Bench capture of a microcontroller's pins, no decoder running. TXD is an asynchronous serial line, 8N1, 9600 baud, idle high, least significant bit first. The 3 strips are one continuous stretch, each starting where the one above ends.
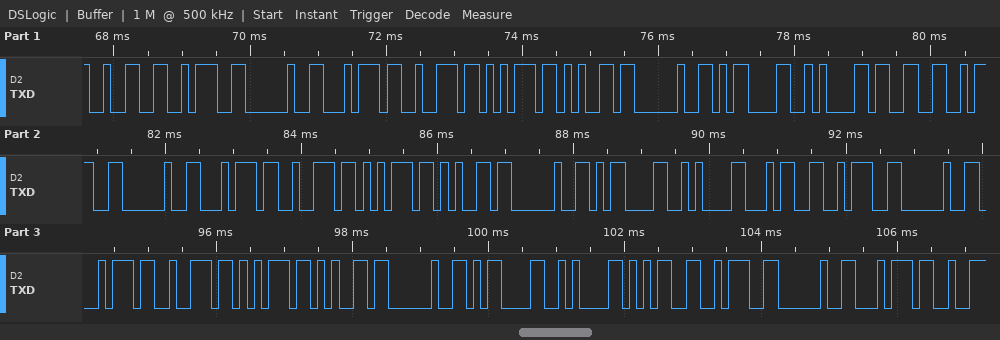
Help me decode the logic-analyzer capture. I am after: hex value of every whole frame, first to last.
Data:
0x32 0x3A 0x20 0x74 0x72 0x75 0x65 0x20 0x0D 0x0A 0x33 0x3A 0x20 0x74 0x72 0x75 0x65 0x20 0x0D 0x0A 0x34 0x3A 0x20 0x74 0x72 0x75 0x65 0x20 0x0D 0x0A 0x35 0x3A 0x20 0x74
